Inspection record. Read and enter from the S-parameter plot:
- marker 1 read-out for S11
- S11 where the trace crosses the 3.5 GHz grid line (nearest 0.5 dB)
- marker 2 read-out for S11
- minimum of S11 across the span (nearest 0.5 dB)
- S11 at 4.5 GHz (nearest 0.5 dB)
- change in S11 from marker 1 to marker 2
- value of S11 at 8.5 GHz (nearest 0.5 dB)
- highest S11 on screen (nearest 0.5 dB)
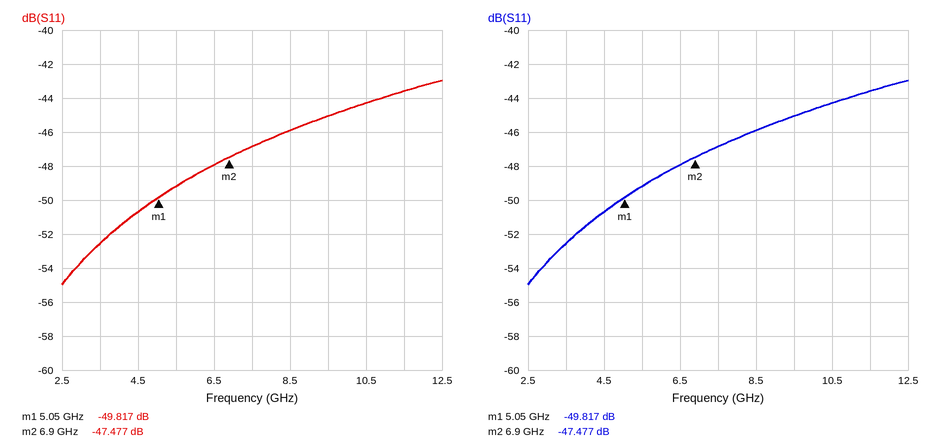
-49.817 dB
-52.5 dB
-47.477 dB
-55.0 dB
-50.5 dB
2.340 dB
-46.0 dB
-43.0 dB
